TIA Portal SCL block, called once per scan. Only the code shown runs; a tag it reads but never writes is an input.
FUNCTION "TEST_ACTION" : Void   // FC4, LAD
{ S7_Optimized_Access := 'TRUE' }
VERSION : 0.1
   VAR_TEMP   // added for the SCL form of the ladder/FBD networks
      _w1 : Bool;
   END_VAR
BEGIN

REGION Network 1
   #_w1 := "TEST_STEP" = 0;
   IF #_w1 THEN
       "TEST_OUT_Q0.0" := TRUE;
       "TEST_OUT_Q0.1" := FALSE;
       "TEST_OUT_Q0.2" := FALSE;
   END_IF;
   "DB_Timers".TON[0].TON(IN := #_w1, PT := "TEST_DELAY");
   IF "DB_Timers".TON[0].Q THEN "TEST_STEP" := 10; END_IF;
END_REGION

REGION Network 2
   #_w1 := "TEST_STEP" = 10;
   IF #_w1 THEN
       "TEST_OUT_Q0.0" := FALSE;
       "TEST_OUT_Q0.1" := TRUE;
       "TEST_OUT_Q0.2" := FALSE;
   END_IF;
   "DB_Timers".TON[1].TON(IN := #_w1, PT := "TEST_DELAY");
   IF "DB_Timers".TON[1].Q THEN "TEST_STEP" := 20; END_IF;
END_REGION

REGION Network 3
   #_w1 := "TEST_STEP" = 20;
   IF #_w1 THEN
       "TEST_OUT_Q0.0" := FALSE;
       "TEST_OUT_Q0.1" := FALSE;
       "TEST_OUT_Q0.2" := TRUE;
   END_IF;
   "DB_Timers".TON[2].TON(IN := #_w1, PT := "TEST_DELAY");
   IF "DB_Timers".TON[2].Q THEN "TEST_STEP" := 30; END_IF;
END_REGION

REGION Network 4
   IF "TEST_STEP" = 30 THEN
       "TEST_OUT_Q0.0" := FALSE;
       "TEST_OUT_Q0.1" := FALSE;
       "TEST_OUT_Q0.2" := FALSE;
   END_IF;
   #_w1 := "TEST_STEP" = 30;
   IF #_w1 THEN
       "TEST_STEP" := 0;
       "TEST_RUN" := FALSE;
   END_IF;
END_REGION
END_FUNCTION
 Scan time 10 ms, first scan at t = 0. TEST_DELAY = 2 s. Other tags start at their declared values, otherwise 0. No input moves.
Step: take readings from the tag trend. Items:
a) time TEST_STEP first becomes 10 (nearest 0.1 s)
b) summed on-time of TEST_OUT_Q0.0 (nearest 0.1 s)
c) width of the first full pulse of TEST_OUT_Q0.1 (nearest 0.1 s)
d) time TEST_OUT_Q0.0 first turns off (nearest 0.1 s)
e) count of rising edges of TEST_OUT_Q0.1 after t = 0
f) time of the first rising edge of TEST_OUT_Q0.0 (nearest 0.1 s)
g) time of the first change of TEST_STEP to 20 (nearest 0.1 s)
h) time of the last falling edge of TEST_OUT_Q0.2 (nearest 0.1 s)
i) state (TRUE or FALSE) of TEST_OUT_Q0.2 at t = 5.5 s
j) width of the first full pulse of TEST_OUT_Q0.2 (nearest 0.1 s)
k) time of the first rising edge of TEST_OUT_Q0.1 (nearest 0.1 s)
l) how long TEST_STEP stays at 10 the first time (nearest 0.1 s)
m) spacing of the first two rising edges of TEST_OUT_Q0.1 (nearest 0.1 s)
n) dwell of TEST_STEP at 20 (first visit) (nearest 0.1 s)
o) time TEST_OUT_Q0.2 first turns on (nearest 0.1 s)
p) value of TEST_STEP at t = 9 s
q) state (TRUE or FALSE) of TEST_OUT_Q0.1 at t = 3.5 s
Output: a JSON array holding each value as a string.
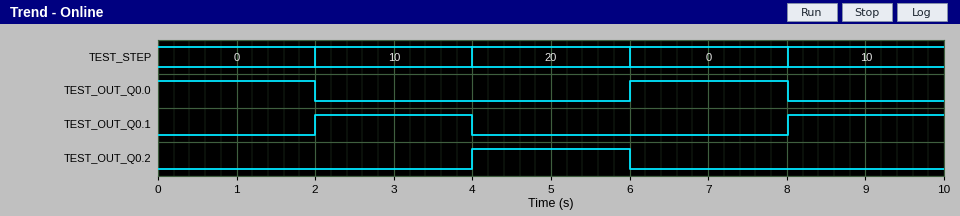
["2.0 s", "4.0 s", "2.0 s", "2.0 s", "2", "6.0 s", "4.0 s", "6.0 s", "TRUE", "2.0 s", "2.0 s", "2.0 s", "6.0 s", "2.0 s", "4.0 s", "10", "TRUE"]
